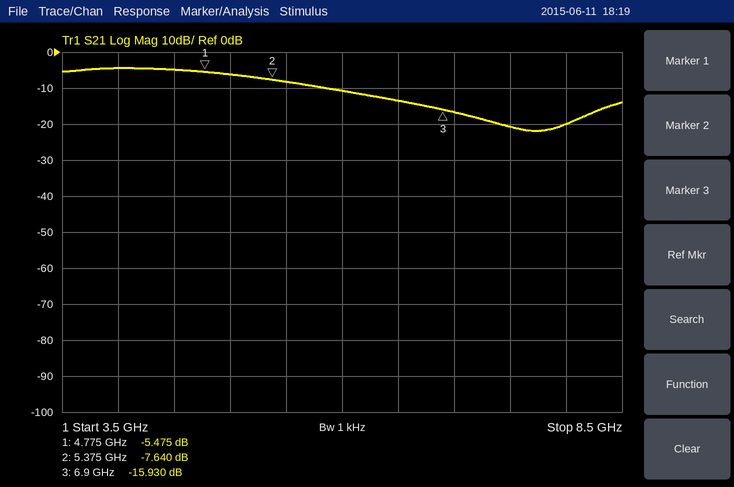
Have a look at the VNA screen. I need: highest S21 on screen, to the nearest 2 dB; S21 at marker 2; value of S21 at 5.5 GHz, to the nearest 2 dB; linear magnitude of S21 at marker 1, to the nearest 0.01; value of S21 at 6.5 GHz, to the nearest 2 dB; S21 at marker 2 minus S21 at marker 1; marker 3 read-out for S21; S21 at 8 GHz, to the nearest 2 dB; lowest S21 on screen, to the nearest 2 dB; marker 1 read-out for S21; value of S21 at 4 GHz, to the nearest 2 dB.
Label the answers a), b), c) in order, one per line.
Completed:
a) -4 dB
b) -7.640 dB
c) -8 dB
d) 0.53
e) -14 dB
f) -2.165 dB
g) -15.930 dB
h) -20 dB
i) -22 dB
j) -5.475 dB
k) -4 dB
